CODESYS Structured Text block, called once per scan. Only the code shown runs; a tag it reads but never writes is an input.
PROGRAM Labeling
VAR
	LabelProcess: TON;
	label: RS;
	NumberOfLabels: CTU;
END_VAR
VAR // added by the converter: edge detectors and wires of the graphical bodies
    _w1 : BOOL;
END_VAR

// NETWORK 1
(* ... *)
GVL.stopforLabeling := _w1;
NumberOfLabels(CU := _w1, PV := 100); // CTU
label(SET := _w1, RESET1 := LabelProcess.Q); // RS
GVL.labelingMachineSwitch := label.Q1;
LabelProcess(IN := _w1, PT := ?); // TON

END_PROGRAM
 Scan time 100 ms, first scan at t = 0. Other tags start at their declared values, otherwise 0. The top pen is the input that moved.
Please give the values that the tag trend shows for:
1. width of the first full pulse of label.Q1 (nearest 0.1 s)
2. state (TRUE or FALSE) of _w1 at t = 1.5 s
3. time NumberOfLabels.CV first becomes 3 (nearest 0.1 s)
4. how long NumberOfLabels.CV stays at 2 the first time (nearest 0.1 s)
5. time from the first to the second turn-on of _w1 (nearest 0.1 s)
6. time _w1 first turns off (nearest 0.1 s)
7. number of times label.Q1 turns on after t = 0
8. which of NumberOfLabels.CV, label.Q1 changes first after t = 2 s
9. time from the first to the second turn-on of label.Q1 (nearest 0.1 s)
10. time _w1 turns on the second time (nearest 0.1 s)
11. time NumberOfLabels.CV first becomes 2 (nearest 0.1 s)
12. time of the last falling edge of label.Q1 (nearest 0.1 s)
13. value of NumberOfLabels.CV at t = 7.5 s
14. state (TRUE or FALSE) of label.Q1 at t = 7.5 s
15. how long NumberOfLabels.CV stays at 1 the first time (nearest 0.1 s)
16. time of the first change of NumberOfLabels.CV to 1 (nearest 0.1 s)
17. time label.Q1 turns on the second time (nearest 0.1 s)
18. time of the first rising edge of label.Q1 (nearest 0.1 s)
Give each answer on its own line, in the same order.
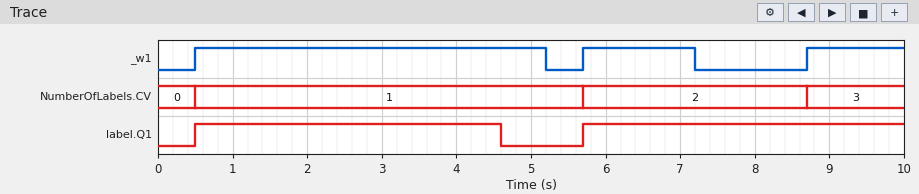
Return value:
4.1 s
TRUE
8.7 s
3.0 s
5.2 s
5.2 s
2
label.Q1
5.2 s
5.7 s
5.7 s
4.6 s
2
TRUE
5.2 s
0.5 s
5.7 s
0.5 s
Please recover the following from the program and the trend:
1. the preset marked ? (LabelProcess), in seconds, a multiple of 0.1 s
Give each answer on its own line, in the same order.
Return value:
4.0 s
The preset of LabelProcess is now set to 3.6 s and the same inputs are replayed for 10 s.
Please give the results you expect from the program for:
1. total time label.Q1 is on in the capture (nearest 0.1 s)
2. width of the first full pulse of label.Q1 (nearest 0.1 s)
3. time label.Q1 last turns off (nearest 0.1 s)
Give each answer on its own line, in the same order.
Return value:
8.0 s
3.7 s
4.2 s
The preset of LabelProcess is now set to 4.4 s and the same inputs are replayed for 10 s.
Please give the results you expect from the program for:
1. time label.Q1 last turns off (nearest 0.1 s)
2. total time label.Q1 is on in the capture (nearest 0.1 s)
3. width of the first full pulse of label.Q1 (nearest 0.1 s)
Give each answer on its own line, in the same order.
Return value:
5.0 s
8.8 s
4.5 s
